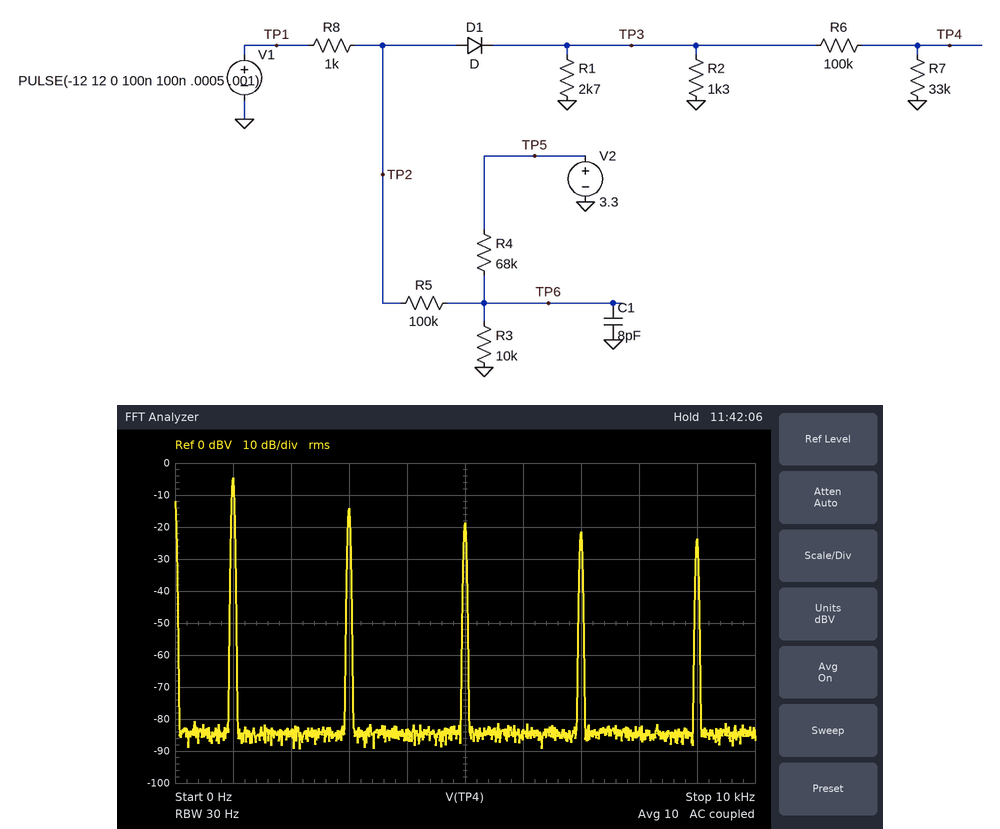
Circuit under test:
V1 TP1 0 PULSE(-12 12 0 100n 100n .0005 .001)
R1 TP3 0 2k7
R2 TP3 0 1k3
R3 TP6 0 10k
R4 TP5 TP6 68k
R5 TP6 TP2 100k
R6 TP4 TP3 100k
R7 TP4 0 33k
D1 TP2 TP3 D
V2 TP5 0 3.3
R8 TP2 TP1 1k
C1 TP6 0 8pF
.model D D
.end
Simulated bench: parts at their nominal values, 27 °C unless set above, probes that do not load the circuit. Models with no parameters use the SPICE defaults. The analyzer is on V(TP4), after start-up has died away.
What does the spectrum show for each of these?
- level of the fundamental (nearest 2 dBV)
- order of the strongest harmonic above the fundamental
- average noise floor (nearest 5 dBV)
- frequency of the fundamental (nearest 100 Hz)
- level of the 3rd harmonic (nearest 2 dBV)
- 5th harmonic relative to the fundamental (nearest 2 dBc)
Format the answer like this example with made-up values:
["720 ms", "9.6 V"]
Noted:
["-4 dBV", "3", "-85 dBV", "1.0 kHz", "-14 dBV", "-14 dBc"]
